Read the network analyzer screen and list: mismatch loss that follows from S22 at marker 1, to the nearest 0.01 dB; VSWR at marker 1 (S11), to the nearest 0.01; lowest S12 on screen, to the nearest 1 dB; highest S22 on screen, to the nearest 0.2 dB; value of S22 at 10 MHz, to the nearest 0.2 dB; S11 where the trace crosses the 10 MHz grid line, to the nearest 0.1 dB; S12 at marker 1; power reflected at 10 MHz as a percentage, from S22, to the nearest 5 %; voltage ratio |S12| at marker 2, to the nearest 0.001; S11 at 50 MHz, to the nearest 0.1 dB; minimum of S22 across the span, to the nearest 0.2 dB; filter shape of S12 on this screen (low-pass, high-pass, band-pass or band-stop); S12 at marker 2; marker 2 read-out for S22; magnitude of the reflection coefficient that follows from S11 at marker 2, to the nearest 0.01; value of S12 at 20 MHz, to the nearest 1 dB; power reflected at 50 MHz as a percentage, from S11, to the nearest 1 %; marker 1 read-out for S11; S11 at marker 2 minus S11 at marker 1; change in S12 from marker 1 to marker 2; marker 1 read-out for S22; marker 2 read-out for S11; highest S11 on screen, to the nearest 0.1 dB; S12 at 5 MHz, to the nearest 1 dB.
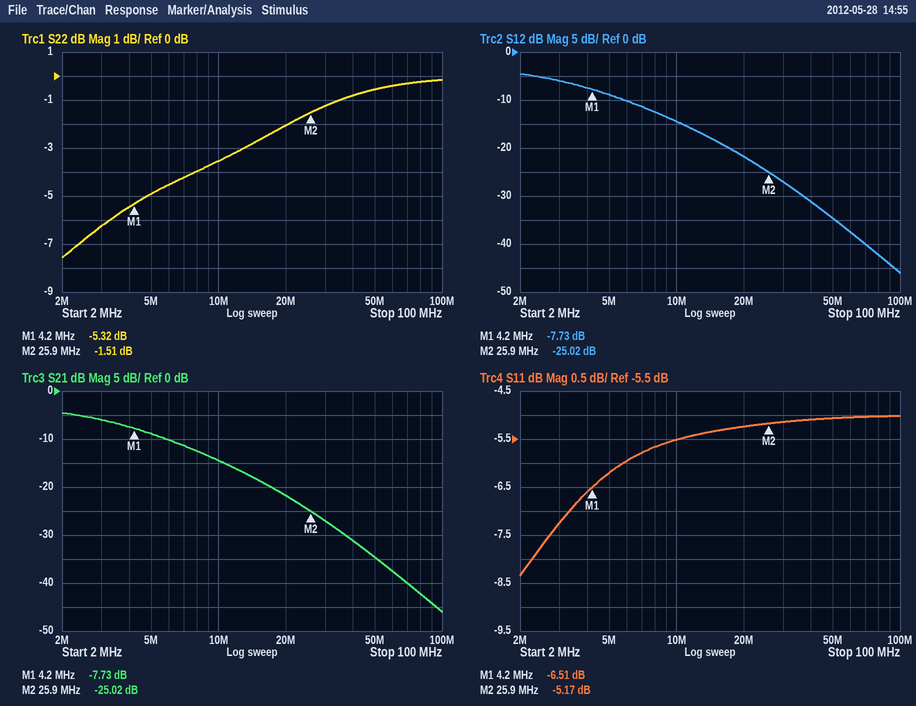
1.51 dB
2.79
-46 dB
-0.2 dB
-3.6 dB
-5.5 dB
-7.73 dB
45 %
0.056
-5.1 dB
-7.6 dB
low-pass
-25.02 dB
-1.51 dB
0.55
-22 dB
31 %
-6.51 dB
1.34 dB
-17.29 dB
-5.32 dB
-5.17 dB
-5.0 dB
-9 dB
